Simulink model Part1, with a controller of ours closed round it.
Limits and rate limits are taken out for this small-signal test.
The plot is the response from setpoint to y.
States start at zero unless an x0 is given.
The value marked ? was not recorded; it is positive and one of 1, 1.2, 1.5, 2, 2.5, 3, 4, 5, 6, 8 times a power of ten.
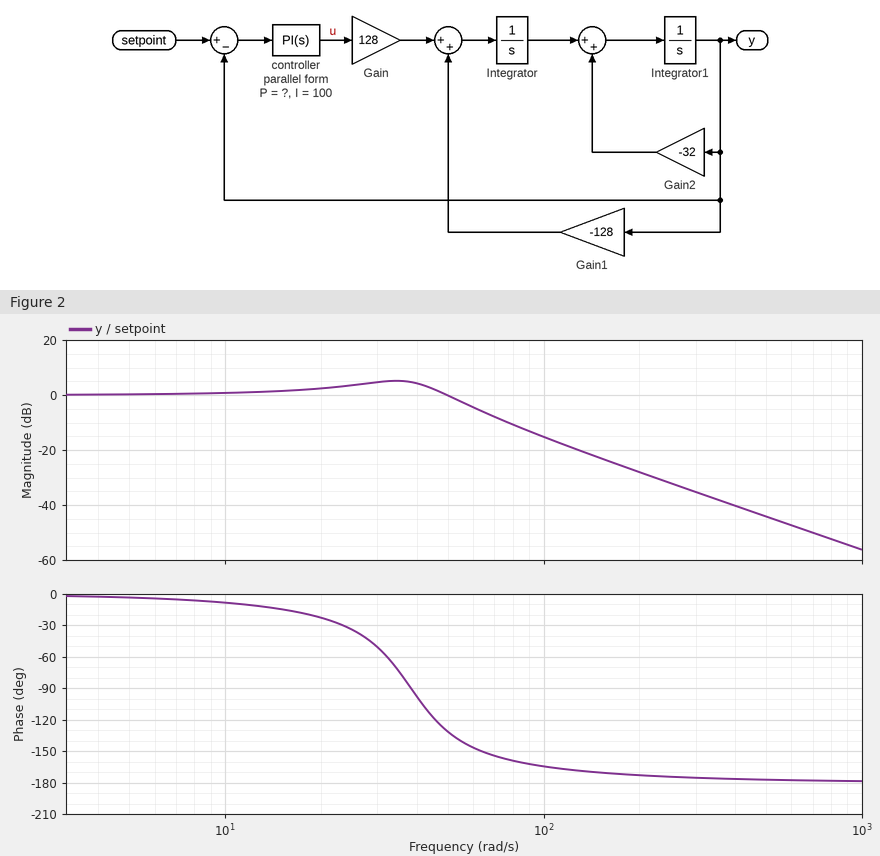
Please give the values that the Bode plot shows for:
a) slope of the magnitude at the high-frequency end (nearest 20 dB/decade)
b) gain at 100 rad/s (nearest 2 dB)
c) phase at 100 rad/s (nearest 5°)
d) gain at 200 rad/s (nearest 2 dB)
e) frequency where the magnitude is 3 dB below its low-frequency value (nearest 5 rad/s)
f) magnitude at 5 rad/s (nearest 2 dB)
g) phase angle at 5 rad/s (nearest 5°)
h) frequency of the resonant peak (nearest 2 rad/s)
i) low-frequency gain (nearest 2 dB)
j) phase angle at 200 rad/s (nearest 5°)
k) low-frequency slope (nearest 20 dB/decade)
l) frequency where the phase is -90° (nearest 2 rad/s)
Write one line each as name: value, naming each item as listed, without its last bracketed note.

slope of the magnitude at the high-frequency end: -40 dB/decade
gain at 100 rad/s: -16 dB
phase at 100 rad/s: -165°
gain at 200 rad/s: -28 dB
frequency where the magnitude is 3 dB below its low-frequency value: 55 rad/s
magnitude at 5 rad/s: 0 dB
phase angle at 5 rad/s: -5°
frequency of the resonant peak: 34 rad/s
low-frequency gain: 0 dB
phase angle at 200 rad/s: -175°
low-frequency slope: 0 dB/decade
frequency where the phase is -90°: 38 rad/s
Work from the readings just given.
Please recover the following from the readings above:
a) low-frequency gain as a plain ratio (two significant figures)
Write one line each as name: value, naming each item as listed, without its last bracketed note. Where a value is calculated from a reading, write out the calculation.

low-frequency gain as a plain ratio: 10^(0 / 20) = 1.0
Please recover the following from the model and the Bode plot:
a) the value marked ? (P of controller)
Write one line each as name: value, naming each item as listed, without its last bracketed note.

the value marked ?: 12
